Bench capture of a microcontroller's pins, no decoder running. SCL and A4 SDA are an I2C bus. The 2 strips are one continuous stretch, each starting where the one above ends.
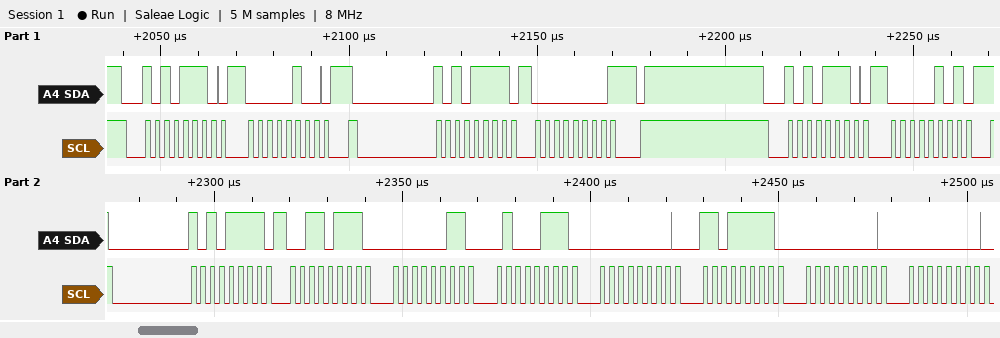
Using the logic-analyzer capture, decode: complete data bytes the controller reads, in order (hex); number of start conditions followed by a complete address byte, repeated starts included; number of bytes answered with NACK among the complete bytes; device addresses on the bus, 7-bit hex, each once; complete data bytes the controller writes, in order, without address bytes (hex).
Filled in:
00 37 03 47 00 DF 00 00
4
1
0x57
04 05
